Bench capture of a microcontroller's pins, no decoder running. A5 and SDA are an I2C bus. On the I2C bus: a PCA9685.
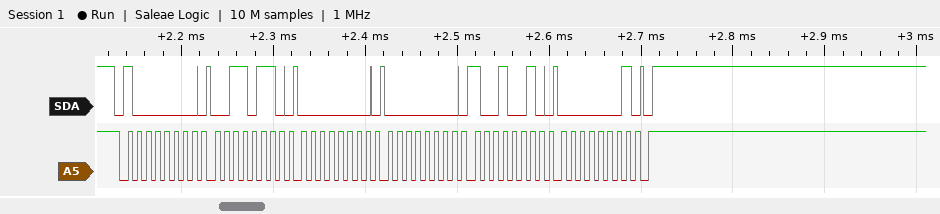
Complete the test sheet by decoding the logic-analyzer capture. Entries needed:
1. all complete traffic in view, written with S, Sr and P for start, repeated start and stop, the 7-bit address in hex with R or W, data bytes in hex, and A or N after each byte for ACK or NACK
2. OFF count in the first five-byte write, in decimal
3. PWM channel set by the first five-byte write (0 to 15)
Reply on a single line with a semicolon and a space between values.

S 40W A 36 A 00 A 00 A 92 A 01 A P; 402; 12
